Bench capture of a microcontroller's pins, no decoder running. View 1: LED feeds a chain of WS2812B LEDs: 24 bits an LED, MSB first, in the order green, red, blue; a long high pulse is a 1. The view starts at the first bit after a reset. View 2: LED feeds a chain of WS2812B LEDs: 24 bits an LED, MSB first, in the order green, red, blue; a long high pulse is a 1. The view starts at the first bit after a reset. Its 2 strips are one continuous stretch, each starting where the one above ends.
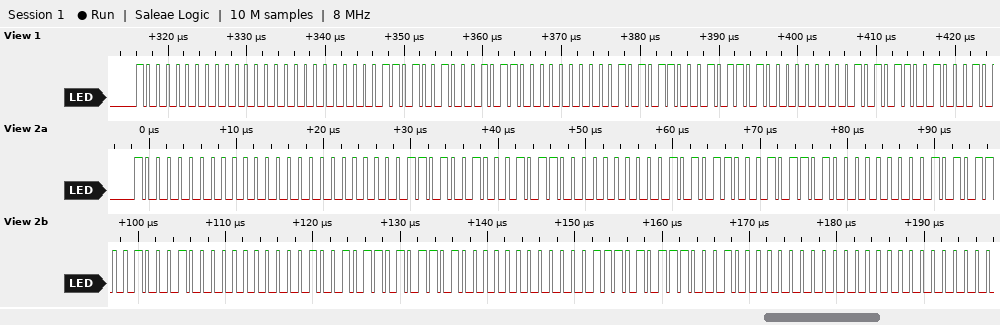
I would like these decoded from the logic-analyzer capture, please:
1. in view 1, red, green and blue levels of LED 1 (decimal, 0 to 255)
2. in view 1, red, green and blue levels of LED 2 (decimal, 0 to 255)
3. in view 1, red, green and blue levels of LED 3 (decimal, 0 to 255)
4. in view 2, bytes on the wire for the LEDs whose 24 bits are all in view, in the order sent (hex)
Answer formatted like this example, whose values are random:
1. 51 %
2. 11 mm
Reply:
1. 0, 128, 0
2. 22, 105, 0
3. 45, 86, 0
4. 80 00 00 69 16 00 56 2D 00 56 44 00 4B 5A 00 1D 71 00
